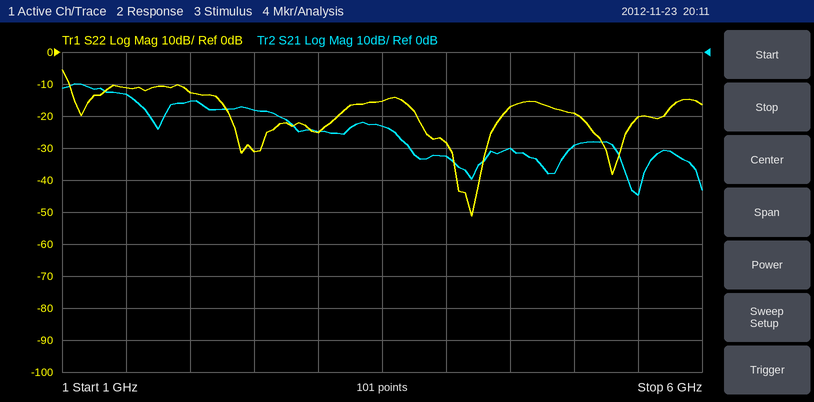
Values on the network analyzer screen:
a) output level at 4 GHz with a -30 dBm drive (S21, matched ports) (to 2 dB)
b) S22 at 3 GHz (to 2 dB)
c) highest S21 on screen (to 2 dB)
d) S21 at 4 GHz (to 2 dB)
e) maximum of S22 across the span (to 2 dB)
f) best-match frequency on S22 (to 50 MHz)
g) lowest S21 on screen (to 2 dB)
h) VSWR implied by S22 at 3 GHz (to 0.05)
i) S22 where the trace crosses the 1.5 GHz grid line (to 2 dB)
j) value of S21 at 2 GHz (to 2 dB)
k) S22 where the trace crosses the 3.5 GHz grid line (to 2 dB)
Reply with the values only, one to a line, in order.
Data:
-62 dBm
-26 dB
-10 dB
-32 dB
-6 dB
4.20 GHz
-44 dB
1.10
-12 dB
-16 dB
-16 dB
